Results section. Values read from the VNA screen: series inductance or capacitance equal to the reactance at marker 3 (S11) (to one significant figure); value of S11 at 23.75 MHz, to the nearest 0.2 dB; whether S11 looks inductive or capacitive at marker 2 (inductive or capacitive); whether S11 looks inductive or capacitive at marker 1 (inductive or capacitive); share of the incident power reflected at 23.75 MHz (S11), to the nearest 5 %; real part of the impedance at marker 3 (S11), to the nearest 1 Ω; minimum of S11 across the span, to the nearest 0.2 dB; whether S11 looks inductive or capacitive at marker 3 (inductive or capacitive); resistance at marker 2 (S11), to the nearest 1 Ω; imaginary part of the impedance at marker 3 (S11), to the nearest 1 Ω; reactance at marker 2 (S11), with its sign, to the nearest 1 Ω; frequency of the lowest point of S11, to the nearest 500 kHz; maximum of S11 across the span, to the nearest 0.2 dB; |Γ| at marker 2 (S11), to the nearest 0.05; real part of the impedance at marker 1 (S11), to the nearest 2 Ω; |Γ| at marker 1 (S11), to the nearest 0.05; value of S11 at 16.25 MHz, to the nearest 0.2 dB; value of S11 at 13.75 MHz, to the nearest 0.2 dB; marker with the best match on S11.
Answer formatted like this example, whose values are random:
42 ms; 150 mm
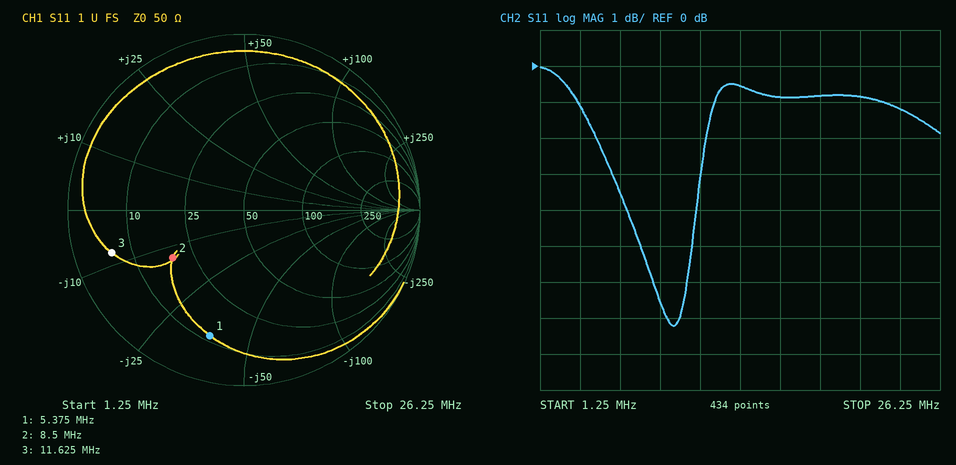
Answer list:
2 nF; -1.2 dB; capacitive; capacitive; 75 %; 6 Ω; -7.2 dB; capacitive; 19 Ω; -8 Ω; -13 Ω; 9.5 MHz; 0.0 dB; 0.50; 12 Ω; 0.75; -0.8 dB; -0.6 dB; marker 2
